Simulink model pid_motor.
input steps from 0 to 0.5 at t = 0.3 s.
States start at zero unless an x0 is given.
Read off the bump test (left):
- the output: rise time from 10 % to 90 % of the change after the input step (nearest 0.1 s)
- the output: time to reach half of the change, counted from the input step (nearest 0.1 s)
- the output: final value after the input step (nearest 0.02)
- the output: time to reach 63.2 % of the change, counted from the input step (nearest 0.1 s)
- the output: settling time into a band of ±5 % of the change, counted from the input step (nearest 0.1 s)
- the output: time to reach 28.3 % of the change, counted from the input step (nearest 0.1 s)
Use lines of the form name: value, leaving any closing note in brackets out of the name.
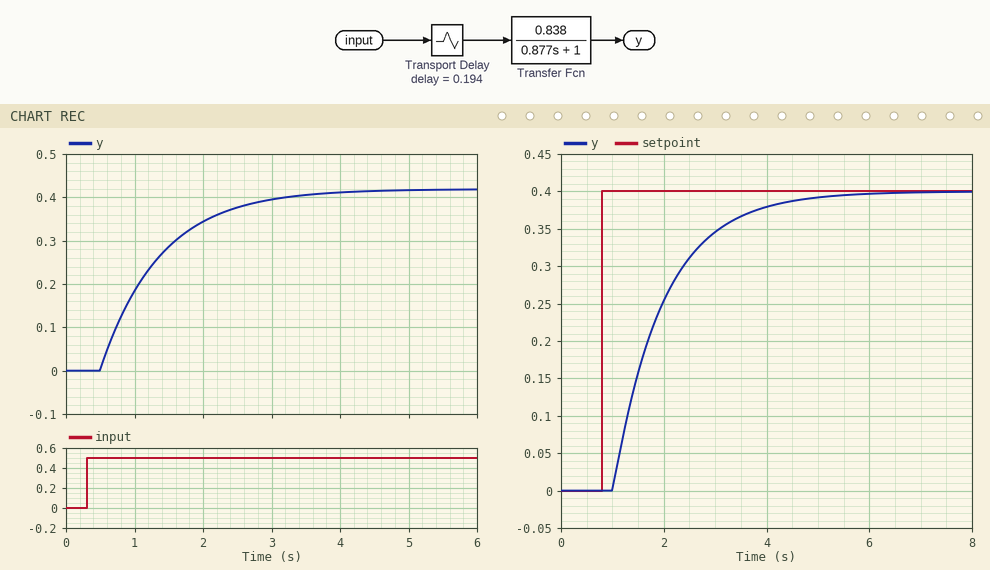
the output: rise time from 10 % to 90 % of the change after the input step: 1.9 s
the output: time to reach half of the change, counted from the input step: 0.8 s
the output: final value after the input step: 0.42
the output: time to reach 63.2 % of the change, counted from the input step: 1.1 s
the output: settling time into a band of ±5 % of the change, counted from the input step: 2.8 s
the output: time to reach 28.3 % of the change, counted from the input step: 0.5 s
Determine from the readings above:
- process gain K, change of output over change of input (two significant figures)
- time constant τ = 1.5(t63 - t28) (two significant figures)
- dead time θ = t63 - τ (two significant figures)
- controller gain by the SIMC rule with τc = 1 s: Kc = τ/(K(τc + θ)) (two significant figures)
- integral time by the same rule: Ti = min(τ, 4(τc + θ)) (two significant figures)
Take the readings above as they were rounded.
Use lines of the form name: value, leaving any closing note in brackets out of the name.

process gain K, change of output over change of input: 0.84
time constant τ = 1.5(t63 - t28): 0.90 s
dead time θ = t63 - τ: 0.20 s
controller gain by the SIMC rule with τc = 1 s: Kc = τ/(K(τc + θ)): 0.89
integral time by the same rule: Ti = min(τ, 4(τc + θ)): 0.90 s
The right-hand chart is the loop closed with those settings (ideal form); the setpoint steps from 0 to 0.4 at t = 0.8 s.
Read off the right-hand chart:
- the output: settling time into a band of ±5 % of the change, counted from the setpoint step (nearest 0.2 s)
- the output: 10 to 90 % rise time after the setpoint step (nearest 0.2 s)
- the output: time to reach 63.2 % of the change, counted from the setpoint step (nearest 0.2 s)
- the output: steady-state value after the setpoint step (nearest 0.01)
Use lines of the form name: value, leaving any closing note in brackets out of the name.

the output: settling time into a band of ±5 % of the change, counted from the setpoint step: 3.2 s
the output: 10 to 90 % rise time after the setpoint step: 2.2 s
the output: time to reach 63.2 % of the change, counted from the setpoint step: 1.2 s
the output: steady-state value after the setpoint step: 0.40
